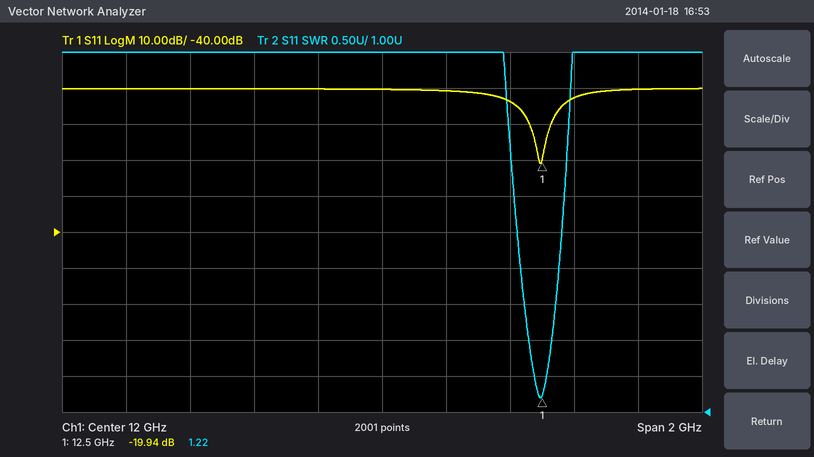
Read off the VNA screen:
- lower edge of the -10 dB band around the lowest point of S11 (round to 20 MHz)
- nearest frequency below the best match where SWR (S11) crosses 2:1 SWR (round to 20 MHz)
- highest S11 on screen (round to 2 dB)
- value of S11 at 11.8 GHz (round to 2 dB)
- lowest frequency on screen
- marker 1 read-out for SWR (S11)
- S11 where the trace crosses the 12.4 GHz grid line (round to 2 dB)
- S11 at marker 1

12.46 GHz
12.46 GHz
0 dB
0 dB
11 GHz
1.22
-4 dB
-19.94 dB
